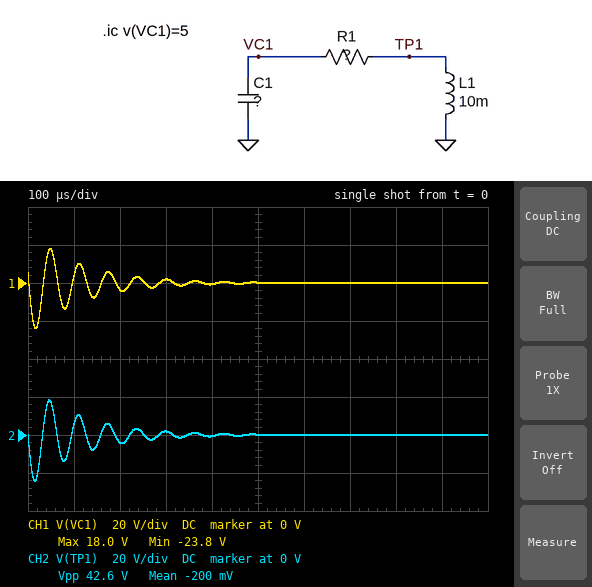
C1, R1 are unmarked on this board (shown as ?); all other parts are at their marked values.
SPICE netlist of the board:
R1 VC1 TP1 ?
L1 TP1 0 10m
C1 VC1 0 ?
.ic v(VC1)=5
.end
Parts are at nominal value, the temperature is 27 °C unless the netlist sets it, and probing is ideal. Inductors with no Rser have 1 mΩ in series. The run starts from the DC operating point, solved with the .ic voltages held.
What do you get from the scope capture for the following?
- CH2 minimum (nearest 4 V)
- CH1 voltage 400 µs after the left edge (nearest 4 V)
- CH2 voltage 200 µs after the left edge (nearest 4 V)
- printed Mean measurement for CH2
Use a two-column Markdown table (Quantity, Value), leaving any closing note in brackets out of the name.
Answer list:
| Quantity | Value |
|---|---|
| CH2 minimum | -24 V |
| CH1 voltage 400 µs after the left edge | 0 V |
| CH2 voltage 200 µs after the left edge | -4 V |
| printed Mean measurement for CH2 | -200 mV |
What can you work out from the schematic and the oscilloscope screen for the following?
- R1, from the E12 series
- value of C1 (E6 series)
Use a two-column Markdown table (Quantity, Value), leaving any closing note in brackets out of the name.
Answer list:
| Quantity | Value |
|---|---|
| R1, from the E12 series | 180 Ω |
| value of C1 | 10 nF |
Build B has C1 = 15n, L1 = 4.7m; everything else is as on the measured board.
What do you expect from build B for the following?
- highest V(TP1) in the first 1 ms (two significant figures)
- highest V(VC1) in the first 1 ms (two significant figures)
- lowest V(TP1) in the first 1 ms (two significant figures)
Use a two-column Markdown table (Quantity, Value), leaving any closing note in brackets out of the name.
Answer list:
| Quantity | Value |
|---|---|
| highest V(TP1) in the first 1 ms | 7.4 V |
| highest V(VC1) in the first 1 ms | 7.0 V |
| lowest V(TP1) in the first 1 ms | -12 V |
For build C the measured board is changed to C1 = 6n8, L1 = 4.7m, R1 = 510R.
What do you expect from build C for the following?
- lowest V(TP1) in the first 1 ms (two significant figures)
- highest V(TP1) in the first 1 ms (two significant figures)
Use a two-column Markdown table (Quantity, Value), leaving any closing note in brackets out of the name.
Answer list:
| Quantity | Value |
|---|---|
| lowest V(TP1) in the first 1 ms | -5.4 V |
| highest V(TP1) in the first 1 ms | 2.0 V |
